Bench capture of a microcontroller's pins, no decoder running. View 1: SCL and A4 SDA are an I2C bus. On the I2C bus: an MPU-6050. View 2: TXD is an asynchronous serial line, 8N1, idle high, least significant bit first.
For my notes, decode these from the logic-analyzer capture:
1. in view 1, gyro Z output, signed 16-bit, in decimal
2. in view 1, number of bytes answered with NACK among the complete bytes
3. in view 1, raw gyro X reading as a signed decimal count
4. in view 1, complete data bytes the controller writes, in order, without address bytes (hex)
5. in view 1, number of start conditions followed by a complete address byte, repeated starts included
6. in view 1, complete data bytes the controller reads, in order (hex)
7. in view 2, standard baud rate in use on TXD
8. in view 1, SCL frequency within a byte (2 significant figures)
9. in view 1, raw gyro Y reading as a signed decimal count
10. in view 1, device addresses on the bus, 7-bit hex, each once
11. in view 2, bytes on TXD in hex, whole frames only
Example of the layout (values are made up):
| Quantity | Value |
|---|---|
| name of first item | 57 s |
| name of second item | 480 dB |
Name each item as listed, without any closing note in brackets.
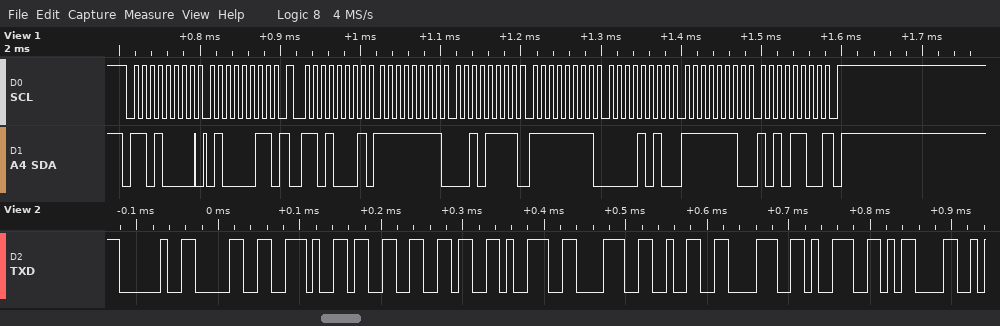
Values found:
| Quantity | Value |
|---|---|
| in view 1, gyro Z output, signed 16-bit, in decimal | -340 |
| in view 1, number of bytes answered with NACK among the complete bytes | 1 |
| in view 1, raw gyro X reading as a signed decimal count | -209 |
| in view 1, complete data bytes the controller writes, in order, without address bytes | 43 |
| in view 1, number of start conditions followed by a complete address byte, repeated starts included | 2 |
| in view 1, complete data bytes the controller reads, in order | FF 2F FF 0A FE AC |
| in view 2, standard baud rate in use on TXD | 115200 baud |
| in view 1, SCL frequency within a byte | 100 kHz |
| in view 1, raw gyro Y reading as a signed decimal count | -246 |
| in view 1, device addresses on the bus, 7-bit hex, each once | 0x68 |
| in view 2, bytes on TXD in hex, whole frames only | 20 30 2E 33 36 39 38 32 38 39 0D |
